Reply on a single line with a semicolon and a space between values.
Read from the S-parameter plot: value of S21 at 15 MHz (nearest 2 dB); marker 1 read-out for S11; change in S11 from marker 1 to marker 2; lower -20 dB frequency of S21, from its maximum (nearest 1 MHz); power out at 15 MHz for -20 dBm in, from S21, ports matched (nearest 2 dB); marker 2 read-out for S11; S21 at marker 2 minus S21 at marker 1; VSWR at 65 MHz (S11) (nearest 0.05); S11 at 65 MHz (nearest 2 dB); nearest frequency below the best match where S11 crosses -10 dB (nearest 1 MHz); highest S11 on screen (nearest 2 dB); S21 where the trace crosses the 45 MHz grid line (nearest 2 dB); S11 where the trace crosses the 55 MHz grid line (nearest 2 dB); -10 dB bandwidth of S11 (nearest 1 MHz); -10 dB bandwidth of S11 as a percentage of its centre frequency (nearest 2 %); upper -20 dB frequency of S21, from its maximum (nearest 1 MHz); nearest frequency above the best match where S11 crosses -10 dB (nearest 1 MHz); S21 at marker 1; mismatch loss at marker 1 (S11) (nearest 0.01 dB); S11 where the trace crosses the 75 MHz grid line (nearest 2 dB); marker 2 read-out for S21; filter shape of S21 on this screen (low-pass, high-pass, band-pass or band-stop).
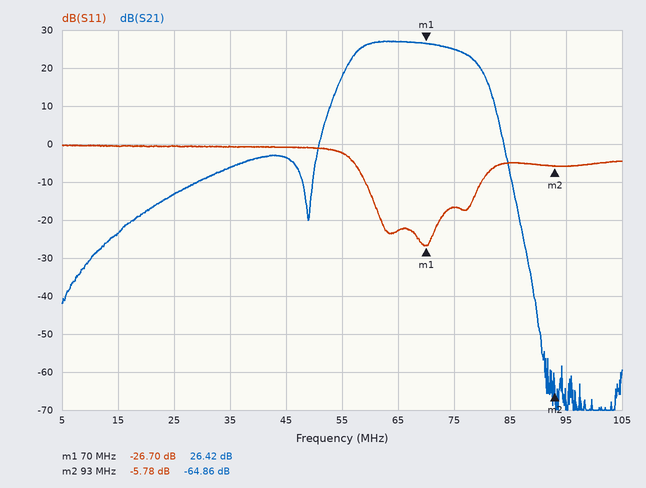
-24 dB; -26.70 dB; 20.92 dB; 52 MHz; -44 dBm; -5.78 dB; -91.28 dB; 1.15; -22 dB; 59 MHz; 0 dB; -4 dB; -2 dB; 21 MHz; 30 %; 83 MHz; 80 MHz; 26.42 dB; 0.01 dB; -16 dB; -64.86 dB; band-pass
